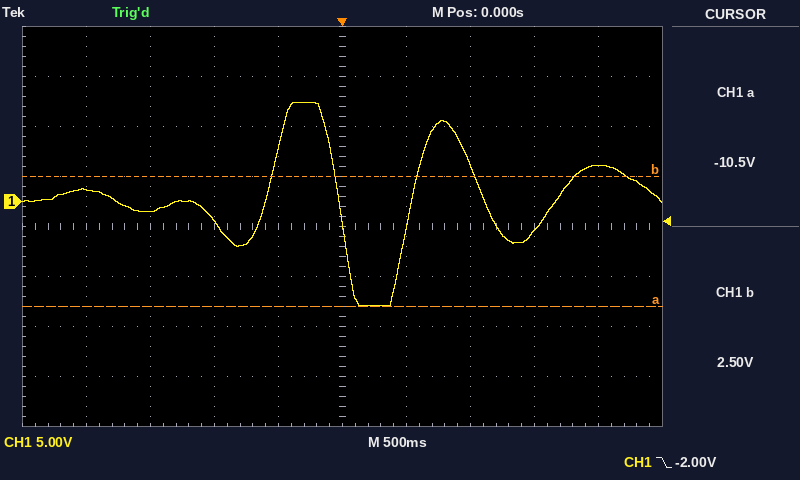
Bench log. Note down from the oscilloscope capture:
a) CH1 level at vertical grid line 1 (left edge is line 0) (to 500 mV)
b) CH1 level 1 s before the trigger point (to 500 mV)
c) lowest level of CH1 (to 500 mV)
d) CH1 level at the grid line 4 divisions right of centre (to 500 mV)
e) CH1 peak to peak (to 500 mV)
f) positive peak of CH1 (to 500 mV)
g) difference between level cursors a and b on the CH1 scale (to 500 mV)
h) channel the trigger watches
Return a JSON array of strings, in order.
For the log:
["1.0 V", "-2.0 V", "-10.5 V", "3.5 V", "20.5 V", "10.0 V", "13.0 V", "CH1"]
